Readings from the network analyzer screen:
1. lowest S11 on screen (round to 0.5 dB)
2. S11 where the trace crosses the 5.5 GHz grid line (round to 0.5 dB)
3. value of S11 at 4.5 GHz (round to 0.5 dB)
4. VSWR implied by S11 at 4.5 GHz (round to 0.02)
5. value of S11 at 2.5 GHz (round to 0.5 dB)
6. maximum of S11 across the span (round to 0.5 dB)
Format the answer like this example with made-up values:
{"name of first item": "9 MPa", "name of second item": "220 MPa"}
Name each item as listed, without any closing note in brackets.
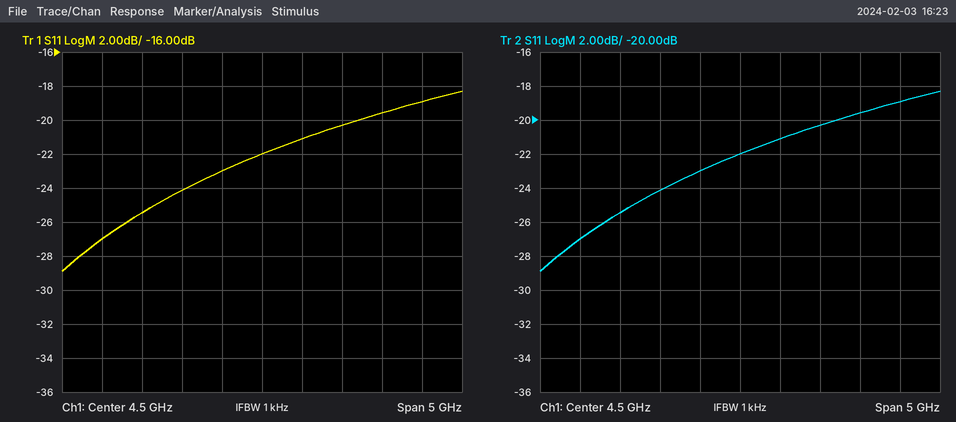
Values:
{"lowest S11 on screen": "-29.0 dB", "S11 where the trace crosses the 5.5 GHz grid line": "-20.5 dB", "value of S11 at 4.5 GHz": "-22.0 dB", "VSWR implied by S11 at 4.5 GHz": "1.18", "value of S11 at 2.5 GHz": "-27.0 dB", "maximum of S11 across the span": "-18.5 dB"}
